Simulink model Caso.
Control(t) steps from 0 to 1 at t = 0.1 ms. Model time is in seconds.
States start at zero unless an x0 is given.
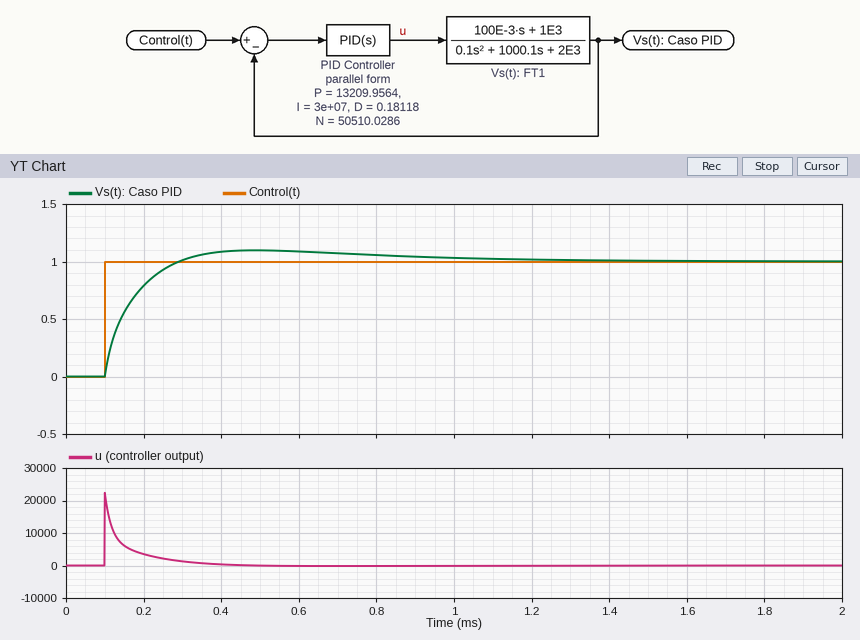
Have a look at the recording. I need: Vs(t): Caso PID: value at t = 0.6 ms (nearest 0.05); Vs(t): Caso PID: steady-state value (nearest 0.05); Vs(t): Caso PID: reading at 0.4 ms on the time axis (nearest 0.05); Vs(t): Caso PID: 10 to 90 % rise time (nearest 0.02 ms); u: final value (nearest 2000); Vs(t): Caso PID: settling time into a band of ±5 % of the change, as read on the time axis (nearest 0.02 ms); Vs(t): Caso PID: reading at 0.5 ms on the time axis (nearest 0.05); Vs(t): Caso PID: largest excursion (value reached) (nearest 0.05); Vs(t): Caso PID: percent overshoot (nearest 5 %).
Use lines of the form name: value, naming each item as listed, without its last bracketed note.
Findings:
Vs(t): Caso PID: value at t = 0.6 ms: 1.10
Vs(t): Caso PID: steady-state value: 1.00
Vs(t): Caso PID: reading at 0.4 ms on the time axis: 1.10
Vs(t): Caso PID: 10 to 90 % rise time: 0.14 ms
u: final value: 0
Vs(t): Caso PID: settling time into a band of ±5 % of the change, as read on the time axis: 0.84 ms
Vs(t): Caso PID: reading at 0.5 ms on the time axis: 1.10
Vs(t): Caso PID: largest excursion (value reached): 1.10
Vs(t): Caso PID: percent overshoot: 10 %
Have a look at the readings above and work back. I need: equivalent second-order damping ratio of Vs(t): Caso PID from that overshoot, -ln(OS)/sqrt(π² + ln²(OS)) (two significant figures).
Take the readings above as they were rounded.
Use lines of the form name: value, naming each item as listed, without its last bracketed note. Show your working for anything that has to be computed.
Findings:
equivalent second-order damping ratio of Vs(t): Caso PID from that overshoot, -ln(OS)/sqrt(π² + ln²(OS)): ln(0.1) = -2.303; 2.303 / sqrt(9.870 + 5.302) = 0.59
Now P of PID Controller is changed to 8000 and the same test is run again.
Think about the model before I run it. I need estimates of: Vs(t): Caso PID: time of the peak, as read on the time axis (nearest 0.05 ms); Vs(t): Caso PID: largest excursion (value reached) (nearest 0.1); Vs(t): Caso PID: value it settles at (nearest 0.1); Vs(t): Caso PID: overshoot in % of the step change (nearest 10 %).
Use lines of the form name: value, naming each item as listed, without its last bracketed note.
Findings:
Vs(t): Caso PID: time of the peak, as read on the time axis: 0.55 ms
Vs(t): Caso PID: largest excursion (value reached): 1.2
Vs(t): Caso PID: value it settles at: 1.0
Vs(t): Caso PID: overshoot in % of the step change: 20 %
